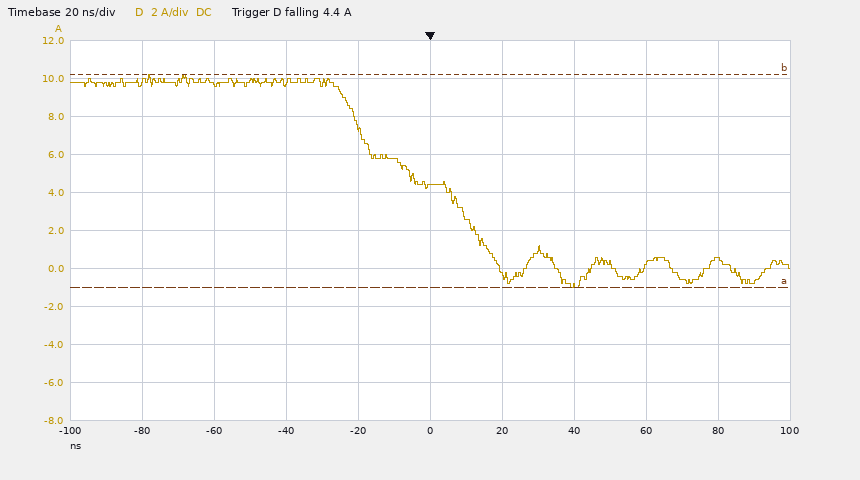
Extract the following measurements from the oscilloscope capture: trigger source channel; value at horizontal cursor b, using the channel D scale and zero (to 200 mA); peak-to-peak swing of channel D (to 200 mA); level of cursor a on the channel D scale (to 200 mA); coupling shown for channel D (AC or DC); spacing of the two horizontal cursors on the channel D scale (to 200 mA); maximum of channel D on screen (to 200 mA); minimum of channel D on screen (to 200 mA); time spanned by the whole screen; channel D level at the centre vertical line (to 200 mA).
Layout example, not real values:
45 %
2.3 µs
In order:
channel D
10.2 A
11.2 A
-1.0 A
DC
11.2 A
10.2 A
-1.0 A
200 ns
4.4 A
